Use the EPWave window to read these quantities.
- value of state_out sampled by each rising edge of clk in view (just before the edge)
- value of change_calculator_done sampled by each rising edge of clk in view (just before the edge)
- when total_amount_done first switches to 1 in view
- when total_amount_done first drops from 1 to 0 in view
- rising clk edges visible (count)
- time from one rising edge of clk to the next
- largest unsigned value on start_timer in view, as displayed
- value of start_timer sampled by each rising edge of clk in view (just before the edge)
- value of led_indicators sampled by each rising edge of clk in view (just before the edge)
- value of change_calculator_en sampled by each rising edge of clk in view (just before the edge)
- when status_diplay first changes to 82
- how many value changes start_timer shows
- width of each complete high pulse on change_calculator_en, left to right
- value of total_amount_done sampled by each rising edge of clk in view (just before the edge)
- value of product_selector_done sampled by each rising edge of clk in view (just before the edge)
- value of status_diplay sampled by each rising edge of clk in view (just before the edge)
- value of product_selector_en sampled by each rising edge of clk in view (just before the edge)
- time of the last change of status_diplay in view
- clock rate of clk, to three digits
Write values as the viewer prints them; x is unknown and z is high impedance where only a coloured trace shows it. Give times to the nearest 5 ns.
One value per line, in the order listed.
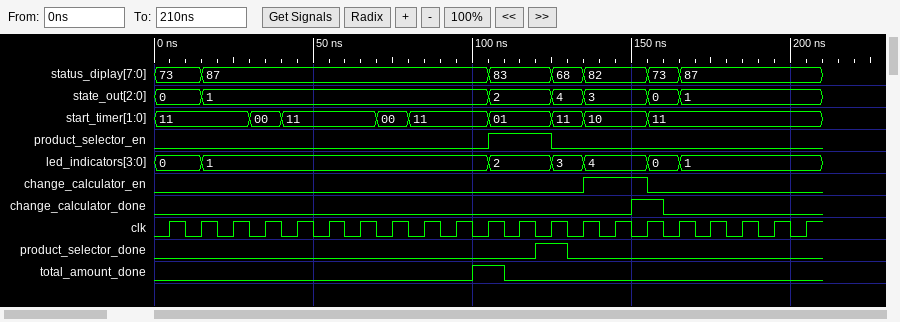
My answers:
0, 0, 1, 1, 1, 1, 1, 1, 1, 1, 1, 2, 2, 4, 3, 3, 0, 1, 1, 1, 1
0 0 0 0 0 0 0 0 0 0 0 0 0 0 0 1 0 0 0 0 0
100 ns
110 ns
21
10 ns
11
11, 11, 11, 00, 11, 11, 11, 00, 11, 11, 11, 01, 01, 11, 10, 10, 11, 11, 11, 11, 11
0, 0, 1, 1, 1, 1, 1, 1, 1, 1, 1, 2, 2, 3, 4, 4, 0, 1, 1, 1, 1
0 0 0 0 0 0 0 0 0 0 0 0 0 0 1 1 0 0 0 0 0
135 ns
8
20 ns
0 0 0 0 0 0 0 0 0 0 1 0 0 0 0 0 0 0 0 0 0
0 0 0 0 0 0 0 0 0 0 0 0 1 0 0 0 0 0 0 0 0
73, 73, 87, 87, 87, 87, 87, 87, 87, 87, 87, 83, 83, 68, 82, 82, 73, 87, 87, 87, 87
0 0 0 0 0 0 0 0 0 0 0 1 1 0 0 0 0 0 0 0 0
165 ns
100 MHz
